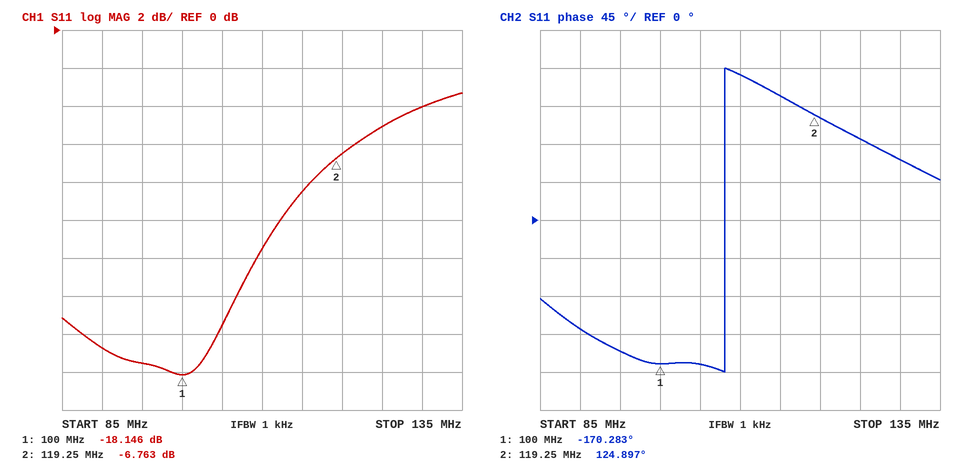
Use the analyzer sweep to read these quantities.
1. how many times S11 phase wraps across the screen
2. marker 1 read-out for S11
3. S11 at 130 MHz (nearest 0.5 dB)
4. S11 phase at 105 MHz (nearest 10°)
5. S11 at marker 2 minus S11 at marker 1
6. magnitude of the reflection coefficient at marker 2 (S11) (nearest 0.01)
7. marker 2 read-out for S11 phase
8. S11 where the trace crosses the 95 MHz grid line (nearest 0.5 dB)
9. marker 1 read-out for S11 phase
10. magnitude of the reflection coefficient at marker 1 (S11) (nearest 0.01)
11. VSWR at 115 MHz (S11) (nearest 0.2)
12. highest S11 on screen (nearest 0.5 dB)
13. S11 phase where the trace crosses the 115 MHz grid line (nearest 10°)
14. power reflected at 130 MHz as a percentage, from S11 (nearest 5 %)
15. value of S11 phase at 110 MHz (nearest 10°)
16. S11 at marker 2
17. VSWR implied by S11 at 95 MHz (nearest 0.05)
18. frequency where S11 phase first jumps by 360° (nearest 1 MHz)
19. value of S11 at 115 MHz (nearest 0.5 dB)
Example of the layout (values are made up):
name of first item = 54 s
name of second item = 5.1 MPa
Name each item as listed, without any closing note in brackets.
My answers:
how many times S11 phase wraps across the screen = 1
marker 1 read-out for S11 = -18.146 dB
S11 at 130 MHz = -4.0 dB
S11 phase at 105 MHz = -170°
S11 at marker 2 minus S11 at marker 1 = 11.383 dB
magnitude of the reflection coefficient at marker 2 (S11) = 0.46
marker 2 read-out for S11 phase = 124.897°
S11 where the trace crosses the 95 MHz grid line = -17.5 dB
marker 1 read-out for S11 phase = -170.283°
magnitude of the reflection coefficient at marker 1 (S11) = 0.12
VSWR at 115 MHz (S11) = 2.2
highest S11 on screen = -3.5 dB
S11 phase where the trace crosses the 115 MHz grid line = 150°
power reflected at 130 MHz as a percentage, from S11 = 40 %
value of S11 phase at 110 MHz = 170°
S11 at marker 2 = -6.763 dB
VSWR implied by S11 at 95 MHz = 1.30
frequency where S11 phase first jumps by 360° = 108 MHz
value of S11 at 115 MHz = -8.5 dB
